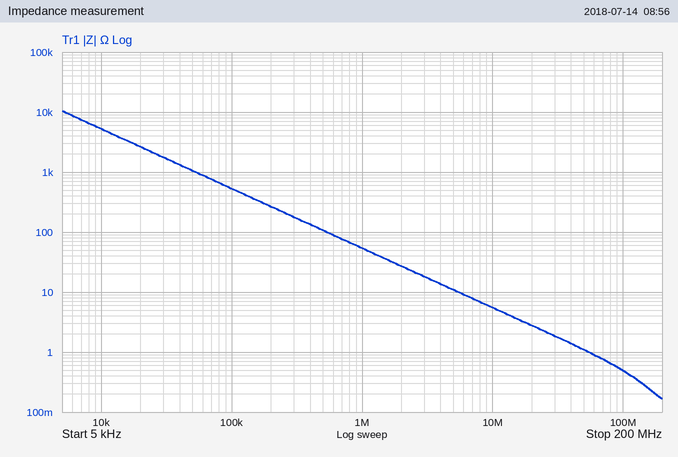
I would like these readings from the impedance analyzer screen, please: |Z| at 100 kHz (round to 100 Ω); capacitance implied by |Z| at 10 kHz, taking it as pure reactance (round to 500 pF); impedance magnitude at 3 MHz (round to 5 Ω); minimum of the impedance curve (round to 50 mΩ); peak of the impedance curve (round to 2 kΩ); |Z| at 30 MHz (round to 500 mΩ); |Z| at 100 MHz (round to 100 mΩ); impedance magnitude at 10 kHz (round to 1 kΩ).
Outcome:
500 Ω
3.0 nF
20 Ω
150 mΩ
10 kΩ
2.0 Ω
500 mΩ
5 kΩ
